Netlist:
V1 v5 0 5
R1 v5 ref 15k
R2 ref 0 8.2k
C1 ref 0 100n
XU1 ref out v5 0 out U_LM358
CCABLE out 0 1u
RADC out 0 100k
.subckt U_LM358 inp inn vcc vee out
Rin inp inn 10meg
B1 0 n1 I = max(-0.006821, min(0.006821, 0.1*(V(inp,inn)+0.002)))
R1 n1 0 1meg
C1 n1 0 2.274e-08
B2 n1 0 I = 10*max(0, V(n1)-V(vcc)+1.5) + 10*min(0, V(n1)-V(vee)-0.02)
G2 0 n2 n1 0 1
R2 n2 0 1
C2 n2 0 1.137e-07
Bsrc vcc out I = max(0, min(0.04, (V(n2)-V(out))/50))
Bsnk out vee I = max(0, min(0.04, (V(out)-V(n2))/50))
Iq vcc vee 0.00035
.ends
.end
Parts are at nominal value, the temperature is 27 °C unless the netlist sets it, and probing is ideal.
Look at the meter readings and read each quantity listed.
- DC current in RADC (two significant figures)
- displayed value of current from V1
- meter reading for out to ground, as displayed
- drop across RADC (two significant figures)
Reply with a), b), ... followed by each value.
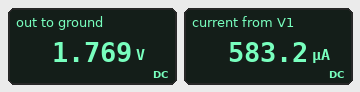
a) 18 µA
b) 583.2 µA
c) 1.769 V
d) 1.8 V
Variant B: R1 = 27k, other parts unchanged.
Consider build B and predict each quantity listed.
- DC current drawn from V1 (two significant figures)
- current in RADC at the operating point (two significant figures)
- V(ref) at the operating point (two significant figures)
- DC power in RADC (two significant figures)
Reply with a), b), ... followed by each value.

a) 500 µA
b) 12 µA
c) 1.2 V
d) 14 µW
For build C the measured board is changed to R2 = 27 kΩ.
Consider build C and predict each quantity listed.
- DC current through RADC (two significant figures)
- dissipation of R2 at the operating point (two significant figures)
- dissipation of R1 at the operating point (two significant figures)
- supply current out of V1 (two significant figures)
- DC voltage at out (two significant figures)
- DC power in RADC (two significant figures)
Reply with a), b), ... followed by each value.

a) 32 µA
b) 380 µW
c) 210 µW
d) 500 µA
e) 3.2 V
f) 100 µW
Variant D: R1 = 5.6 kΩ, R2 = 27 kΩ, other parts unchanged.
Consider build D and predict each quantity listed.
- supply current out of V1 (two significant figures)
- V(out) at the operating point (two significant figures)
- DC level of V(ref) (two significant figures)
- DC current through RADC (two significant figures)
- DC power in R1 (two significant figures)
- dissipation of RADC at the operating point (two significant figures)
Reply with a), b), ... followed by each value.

a) 540 µA
b) 3.5 V
c) 4.1 V
d) 35 µA
e) 130 µW
f) 120 µW
